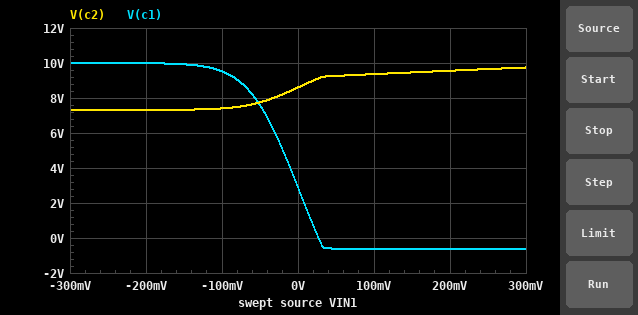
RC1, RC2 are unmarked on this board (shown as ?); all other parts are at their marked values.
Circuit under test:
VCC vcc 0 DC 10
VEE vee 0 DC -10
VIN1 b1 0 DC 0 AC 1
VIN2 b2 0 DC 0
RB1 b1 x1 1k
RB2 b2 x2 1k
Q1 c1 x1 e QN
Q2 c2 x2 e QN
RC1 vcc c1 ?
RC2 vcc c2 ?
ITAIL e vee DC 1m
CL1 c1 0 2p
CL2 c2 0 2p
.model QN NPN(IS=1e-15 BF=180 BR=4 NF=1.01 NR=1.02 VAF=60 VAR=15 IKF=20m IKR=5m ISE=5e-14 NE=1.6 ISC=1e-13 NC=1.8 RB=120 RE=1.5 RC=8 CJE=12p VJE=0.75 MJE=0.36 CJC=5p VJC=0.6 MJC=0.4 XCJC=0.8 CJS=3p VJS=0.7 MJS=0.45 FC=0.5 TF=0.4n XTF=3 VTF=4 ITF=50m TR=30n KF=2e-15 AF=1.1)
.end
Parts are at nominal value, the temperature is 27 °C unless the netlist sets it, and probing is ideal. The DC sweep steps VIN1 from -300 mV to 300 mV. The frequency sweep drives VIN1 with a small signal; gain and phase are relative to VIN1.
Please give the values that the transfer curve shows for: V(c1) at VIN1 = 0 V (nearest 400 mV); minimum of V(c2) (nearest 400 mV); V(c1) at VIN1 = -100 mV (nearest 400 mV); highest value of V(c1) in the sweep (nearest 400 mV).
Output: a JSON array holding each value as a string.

["2.8 V", "7.2 V", "9.6 V", "10.0 V"]
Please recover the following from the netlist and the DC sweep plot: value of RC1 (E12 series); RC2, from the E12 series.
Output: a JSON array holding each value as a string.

["15 kΩ", "2.7 kΩ"]
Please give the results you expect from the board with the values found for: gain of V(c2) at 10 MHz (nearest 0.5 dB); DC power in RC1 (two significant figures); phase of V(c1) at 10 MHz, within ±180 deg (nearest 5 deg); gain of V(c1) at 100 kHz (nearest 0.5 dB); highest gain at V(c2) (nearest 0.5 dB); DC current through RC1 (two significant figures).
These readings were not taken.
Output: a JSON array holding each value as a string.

["7.5 dB", "3.4 mW", "65 deg", "40.5 dB", "26.0 dB", "470 µA"]
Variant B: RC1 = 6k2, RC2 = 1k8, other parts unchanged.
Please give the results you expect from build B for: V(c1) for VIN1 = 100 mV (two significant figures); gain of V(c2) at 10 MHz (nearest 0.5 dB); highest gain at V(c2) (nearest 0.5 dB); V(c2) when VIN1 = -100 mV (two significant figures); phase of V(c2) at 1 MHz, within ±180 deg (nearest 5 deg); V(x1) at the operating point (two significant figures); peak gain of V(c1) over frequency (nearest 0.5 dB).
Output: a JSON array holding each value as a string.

["4.1 V", "6.0 dB", "23.0 dB", "8.3 V", "-40 deg", "-3.8 mV", "33.5 dB"]
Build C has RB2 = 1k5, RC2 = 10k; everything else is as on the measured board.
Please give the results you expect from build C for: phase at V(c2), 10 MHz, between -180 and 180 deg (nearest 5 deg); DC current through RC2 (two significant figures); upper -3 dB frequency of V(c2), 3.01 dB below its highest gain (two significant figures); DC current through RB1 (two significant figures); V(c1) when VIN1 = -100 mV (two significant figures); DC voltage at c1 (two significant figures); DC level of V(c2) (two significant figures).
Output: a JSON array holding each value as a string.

["-90 deg", "490 µA", "260 kHz", "4.1 µA", "9.4 V", "2.5 V", "5.1 V"]
